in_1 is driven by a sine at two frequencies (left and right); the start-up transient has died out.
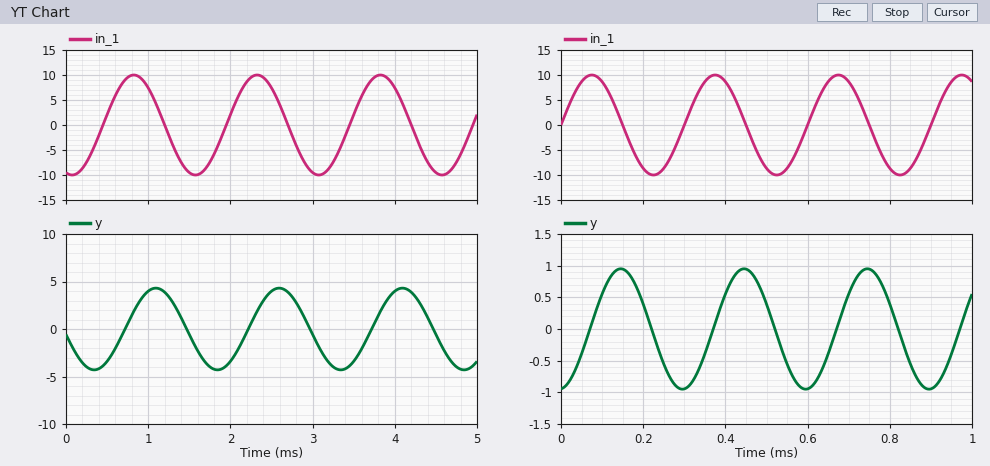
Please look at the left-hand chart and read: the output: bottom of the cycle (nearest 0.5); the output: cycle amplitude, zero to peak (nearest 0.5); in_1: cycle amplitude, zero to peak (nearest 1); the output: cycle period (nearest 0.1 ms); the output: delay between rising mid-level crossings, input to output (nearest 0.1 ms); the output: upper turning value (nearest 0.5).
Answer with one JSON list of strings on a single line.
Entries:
["-4.5", "4.5", "10", "1.5 ms", "0.3 ms", "4.5"]
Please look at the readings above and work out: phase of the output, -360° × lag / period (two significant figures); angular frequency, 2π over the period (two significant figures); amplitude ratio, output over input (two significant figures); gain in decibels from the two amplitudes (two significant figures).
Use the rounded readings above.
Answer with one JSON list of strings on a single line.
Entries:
["-72°", "4.2 rad/ms", "0.45", "-6.9 dB"]
